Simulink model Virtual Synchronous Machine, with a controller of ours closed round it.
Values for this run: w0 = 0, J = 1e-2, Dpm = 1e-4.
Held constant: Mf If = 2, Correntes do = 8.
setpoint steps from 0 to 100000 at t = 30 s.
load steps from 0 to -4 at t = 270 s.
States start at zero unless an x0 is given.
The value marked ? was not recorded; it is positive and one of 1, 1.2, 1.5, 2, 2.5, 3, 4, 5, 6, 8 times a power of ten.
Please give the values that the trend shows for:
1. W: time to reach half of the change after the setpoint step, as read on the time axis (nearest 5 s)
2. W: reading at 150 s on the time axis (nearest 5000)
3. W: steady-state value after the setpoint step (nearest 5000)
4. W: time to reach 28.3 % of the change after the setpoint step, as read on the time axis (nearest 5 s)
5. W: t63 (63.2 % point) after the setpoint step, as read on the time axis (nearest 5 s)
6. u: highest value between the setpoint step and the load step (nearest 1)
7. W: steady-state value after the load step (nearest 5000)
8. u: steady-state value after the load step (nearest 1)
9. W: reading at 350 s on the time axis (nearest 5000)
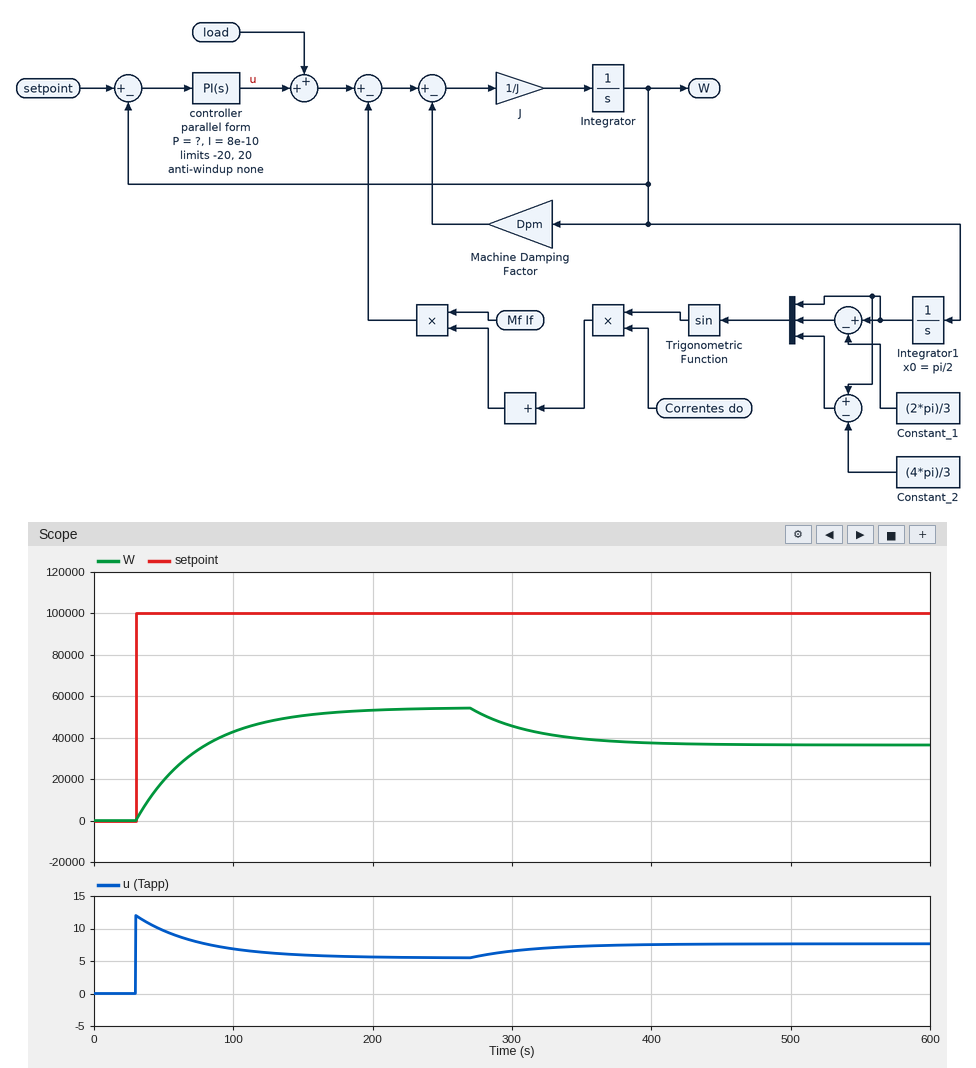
60 s
50000
55000
45 s
75 s
12
35000
8
40000
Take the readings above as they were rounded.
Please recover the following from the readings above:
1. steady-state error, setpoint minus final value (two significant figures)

45000
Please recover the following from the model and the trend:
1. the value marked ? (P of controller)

0.00012
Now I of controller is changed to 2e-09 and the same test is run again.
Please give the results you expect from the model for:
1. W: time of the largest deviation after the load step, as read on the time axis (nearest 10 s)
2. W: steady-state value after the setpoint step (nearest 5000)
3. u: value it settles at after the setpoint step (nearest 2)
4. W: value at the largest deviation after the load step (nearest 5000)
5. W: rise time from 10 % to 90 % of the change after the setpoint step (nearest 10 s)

570 s
55000
6
35000
110 s
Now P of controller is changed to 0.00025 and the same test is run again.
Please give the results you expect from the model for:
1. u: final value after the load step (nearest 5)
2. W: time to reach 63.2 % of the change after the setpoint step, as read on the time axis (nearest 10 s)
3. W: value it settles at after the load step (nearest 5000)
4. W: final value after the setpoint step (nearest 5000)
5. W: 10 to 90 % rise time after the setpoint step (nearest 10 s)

10
60 s
60000
70000
60 s
